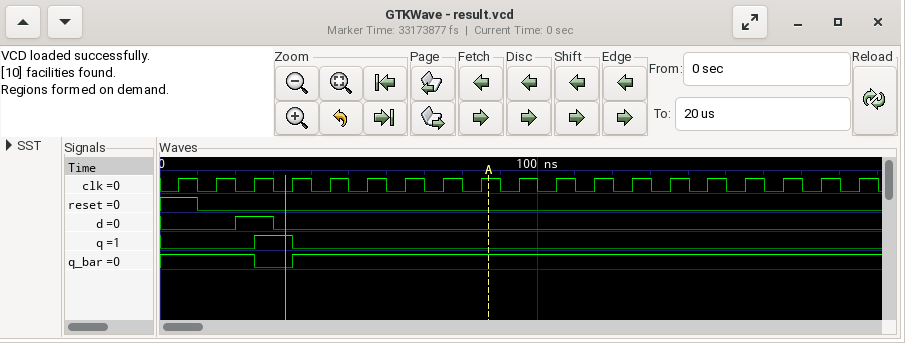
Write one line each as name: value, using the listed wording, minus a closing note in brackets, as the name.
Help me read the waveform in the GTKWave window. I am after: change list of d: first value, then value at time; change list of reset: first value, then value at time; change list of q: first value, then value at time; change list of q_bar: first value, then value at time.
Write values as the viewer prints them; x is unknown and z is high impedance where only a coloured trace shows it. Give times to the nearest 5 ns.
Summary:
change list of d: first value, then value at time: 0, 1 at 20 ns, 0 at 30 ns
change list of reset: first value, then value at time: 1, 0 at 10 ns
change list of q: first value, then value at time: 0, 1 at 25 ns, 0 at 35 ns
change list of q_bar: first value, then value at time: 1, 0 at 25 ns, 1 at 35 ns
